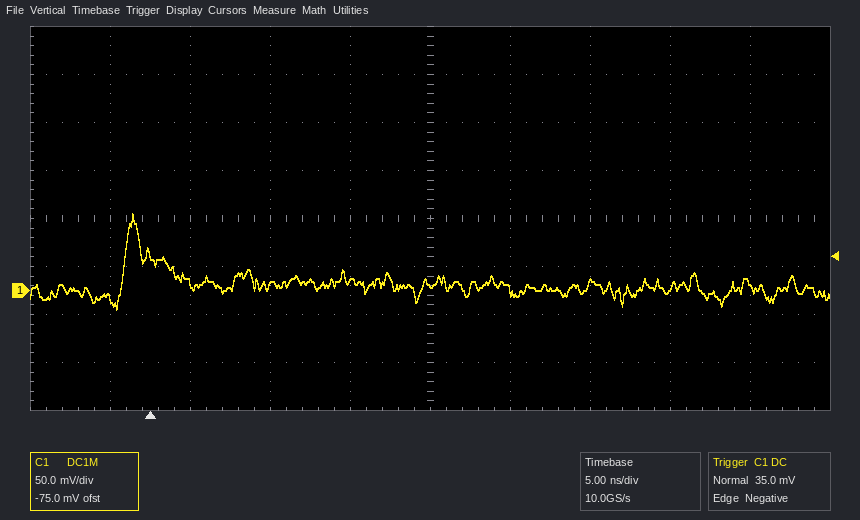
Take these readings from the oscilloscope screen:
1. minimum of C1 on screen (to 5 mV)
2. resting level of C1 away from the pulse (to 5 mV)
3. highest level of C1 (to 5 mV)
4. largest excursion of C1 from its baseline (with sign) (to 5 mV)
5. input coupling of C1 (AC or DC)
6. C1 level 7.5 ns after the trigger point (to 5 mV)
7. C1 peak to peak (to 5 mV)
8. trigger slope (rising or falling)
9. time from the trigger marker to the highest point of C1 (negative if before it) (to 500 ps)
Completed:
-20 mV
5 mV
80 mV
+75 mV
DC
5 mV
100 mV
falling
-1.0 ns
